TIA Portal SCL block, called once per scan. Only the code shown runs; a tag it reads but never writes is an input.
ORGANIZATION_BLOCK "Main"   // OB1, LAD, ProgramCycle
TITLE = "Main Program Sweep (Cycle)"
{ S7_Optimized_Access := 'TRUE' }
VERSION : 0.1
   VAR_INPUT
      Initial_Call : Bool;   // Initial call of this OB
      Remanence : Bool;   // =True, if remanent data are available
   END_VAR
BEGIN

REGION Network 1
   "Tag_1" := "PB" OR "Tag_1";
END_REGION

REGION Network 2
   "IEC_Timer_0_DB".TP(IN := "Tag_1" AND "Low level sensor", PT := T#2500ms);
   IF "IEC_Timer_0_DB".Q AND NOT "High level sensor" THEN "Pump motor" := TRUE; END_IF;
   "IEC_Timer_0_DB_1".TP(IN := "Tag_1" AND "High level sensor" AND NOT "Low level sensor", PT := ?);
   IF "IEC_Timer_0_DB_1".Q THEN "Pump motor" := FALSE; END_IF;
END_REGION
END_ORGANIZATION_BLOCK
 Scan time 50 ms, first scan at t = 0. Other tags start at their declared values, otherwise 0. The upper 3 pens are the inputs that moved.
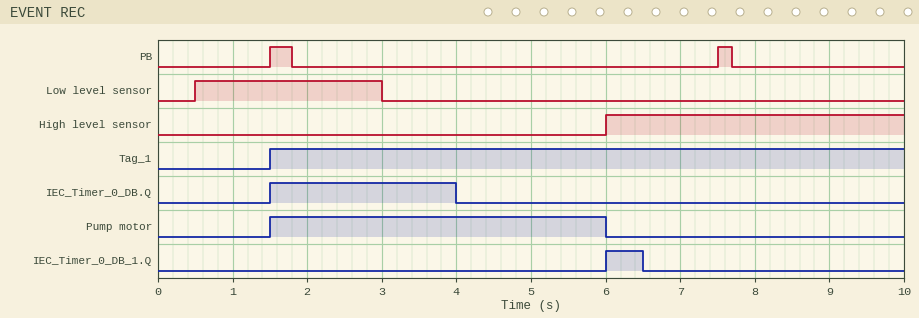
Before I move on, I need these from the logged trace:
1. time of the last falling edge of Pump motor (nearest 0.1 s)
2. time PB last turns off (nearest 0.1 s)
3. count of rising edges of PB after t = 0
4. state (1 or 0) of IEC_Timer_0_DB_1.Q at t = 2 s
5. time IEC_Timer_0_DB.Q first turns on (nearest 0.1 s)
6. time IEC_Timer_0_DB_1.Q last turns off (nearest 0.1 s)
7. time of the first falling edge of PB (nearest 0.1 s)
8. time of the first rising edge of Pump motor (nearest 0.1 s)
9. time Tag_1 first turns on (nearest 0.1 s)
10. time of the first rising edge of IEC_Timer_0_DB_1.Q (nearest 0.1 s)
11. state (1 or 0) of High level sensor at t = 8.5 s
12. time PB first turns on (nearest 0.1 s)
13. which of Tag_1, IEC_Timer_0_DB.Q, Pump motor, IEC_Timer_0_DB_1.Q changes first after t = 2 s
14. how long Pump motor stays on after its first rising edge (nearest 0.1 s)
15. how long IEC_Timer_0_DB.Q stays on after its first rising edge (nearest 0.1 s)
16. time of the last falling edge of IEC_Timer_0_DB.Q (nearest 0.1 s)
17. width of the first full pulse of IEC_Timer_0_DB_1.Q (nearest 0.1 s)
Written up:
6.0 s
7.7 s
2
0
1.5 s
6.5 s
1.8 s
1.5 s
1.5 s
6.0 s
1
1.5 s
IEC_Timer_0_DB.Q
4.5 s
2.5 s
4.0 s
0.5 s
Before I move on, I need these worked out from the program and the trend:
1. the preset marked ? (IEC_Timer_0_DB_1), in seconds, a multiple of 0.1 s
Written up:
0.5 s
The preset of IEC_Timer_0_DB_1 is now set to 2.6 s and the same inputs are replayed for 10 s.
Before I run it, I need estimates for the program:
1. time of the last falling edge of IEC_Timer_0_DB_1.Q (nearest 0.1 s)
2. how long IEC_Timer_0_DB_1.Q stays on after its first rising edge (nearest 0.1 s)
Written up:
8.6 s
2.6 s
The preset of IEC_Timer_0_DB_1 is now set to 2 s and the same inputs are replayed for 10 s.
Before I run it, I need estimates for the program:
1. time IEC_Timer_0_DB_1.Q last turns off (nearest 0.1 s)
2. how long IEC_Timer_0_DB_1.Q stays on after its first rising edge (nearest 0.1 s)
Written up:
8.0 s
2.0 s
